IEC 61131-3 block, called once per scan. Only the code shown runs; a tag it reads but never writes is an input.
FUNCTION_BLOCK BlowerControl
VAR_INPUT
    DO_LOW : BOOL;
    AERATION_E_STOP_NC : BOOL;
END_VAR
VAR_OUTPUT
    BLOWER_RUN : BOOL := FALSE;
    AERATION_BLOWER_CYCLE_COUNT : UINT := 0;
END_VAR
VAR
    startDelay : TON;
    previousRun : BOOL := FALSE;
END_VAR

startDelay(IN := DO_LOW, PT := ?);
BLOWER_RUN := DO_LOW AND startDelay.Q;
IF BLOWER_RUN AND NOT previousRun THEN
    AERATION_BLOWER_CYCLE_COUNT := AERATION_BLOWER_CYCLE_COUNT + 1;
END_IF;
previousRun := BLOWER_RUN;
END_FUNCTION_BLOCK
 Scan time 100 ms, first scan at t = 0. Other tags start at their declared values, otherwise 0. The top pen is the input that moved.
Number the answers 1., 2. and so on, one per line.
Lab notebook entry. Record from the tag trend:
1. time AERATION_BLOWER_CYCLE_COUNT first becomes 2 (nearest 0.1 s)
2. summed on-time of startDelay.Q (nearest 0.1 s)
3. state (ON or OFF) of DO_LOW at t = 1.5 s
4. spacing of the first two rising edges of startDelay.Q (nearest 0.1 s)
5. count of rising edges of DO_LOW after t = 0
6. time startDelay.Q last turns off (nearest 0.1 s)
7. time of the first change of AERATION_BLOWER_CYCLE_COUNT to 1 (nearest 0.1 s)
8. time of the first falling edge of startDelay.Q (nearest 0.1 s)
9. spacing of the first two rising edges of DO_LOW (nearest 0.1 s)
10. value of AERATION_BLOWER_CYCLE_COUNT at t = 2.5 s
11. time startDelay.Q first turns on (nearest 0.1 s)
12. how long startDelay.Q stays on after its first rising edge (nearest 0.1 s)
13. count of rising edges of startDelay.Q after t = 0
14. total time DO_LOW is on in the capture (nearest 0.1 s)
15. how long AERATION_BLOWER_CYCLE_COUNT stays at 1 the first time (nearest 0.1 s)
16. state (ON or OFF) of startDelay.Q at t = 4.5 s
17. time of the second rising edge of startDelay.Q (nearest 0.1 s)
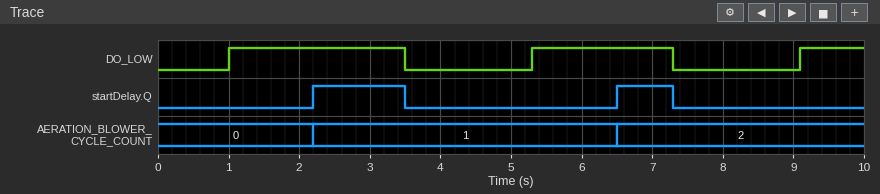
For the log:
1. 6.5 s
2. 2.1 s
3. ON
4. 4.3 s
5. 3
6. 7.3 s
7. 2.2 s
8. 3.5 s
9. 4.3 s
10. 1
11. 2.2 s
12. 1.3 s
13. 2
14. 5.4 s
15. 4.3 s
16. OFF
17. 6.5 s
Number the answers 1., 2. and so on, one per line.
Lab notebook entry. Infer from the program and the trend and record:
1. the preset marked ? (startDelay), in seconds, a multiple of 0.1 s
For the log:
1. 1.2 s
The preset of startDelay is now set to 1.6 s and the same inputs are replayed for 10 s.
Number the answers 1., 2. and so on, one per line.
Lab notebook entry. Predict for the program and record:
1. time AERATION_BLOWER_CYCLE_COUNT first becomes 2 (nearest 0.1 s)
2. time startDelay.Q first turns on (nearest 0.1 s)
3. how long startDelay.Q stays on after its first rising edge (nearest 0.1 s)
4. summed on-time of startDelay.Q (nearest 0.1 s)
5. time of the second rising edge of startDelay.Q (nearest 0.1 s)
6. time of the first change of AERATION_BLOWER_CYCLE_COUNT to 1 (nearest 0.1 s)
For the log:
1. 6.9 s
2. 2.6 s
3. 0.9 s
4. 1.3 s
5. 6.9 s
6. 2.6 s
